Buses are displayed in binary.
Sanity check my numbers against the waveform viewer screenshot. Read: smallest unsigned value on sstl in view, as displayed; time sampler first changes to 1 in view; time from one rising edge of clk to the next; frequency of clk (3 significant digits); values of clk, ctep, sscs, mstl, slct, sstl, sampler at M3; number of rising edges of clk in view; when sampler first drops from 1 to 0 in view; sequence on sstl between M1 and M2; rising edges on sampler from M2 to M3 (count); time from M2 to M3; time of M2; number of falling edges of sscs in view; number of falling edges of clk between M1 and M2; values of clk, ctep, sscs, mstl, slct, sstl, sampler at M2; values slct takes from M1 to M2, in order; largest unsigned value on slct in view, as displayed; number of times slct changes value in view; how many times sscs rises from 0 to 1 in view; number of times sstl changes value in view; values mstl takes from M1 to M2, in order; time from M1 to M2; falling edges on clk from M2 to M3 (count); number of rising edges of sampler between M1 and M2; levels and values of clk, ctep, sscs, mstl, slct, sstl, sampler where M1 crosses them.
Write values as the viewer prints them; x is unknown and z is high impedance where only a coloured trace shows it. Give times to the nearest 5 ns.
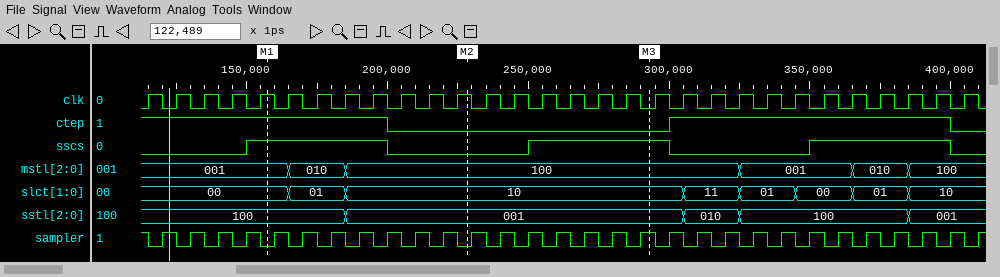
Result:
001
120 ns
10 ns
100 MHz
clk=0, ctep=0, sscs=1, mstl=100, slct=10, sstl=001, sampler=1
30
115 ns
100, 001
7
65 ns
230 ns
3
7
clk=1, ctep=0, sscs=0, mstl=100, slct=10, sstl=001, sampler=0
00, 01, 10
11
7
3
4
001, 010, 100
70 ns
7
7
clk=1, ctep=1, sscs=1, mstl=001, slct=00, sstl=100, sampler=0
